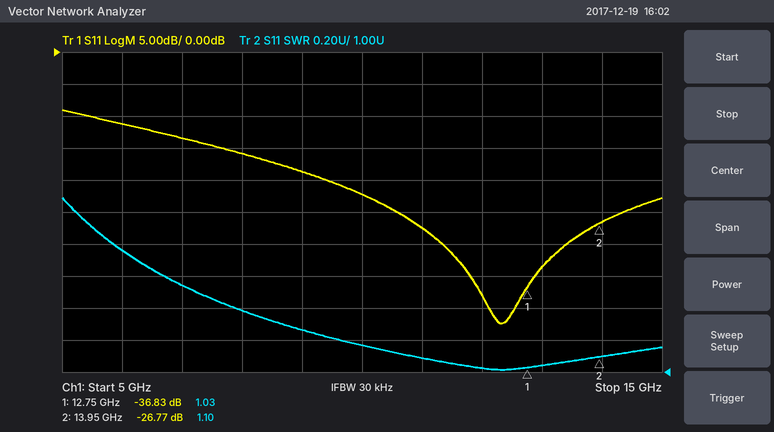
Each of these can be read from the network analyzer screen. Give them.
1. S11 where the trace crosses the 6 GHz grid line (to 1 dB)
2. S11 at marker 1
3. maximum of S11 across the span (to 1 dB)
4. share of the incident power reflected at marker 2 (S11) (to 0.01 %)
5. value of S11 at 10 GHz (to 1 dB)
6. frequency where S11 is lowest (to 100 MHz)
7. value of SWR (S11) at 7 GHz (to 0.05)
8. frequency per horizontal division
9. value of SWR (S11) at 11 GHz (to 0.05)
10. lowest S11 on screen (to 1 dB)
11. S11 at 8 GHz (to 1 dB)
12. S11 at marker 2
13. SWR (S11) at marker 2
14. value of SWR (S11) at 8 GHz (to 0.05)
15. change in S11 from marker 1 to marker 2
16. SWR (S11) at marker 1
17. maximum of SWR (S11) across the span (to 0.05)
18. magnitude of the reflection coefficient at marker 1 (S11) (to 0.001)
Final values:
-11 dB
-36.83 dB
-9 dB
0.21 %
-22 dB
12.3 GHz
1.55
1 GHz
1.10
-42 dB
-16 dB
-26.77 dB
1.10
1.40
10.06 dB
1.03
2.10
0.014
